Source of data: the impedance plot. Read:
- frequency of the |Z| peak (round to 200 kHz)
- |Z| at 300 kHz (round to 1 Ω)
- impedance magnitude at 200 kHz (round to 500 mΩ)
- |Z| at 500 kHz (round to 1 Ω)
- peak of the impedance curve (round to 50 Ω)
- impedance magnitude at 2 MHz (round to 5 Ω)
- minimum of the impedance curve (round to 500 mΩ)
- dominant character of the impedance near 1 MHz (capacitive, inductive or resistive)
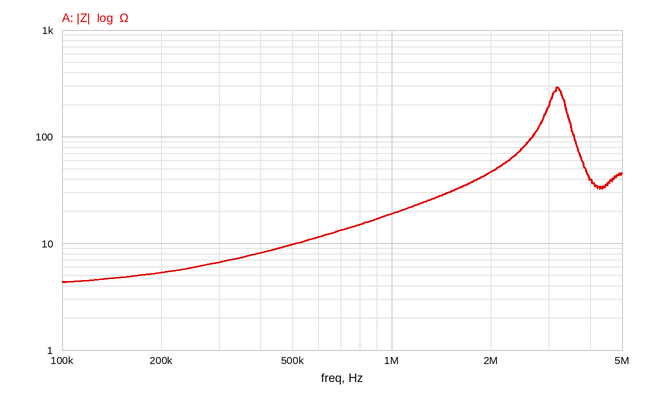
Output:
3.2 MHz
7 Ω
5.5 Ω
10 Ω
300 Ω
45 Ω
4.5 Ω
inductive
